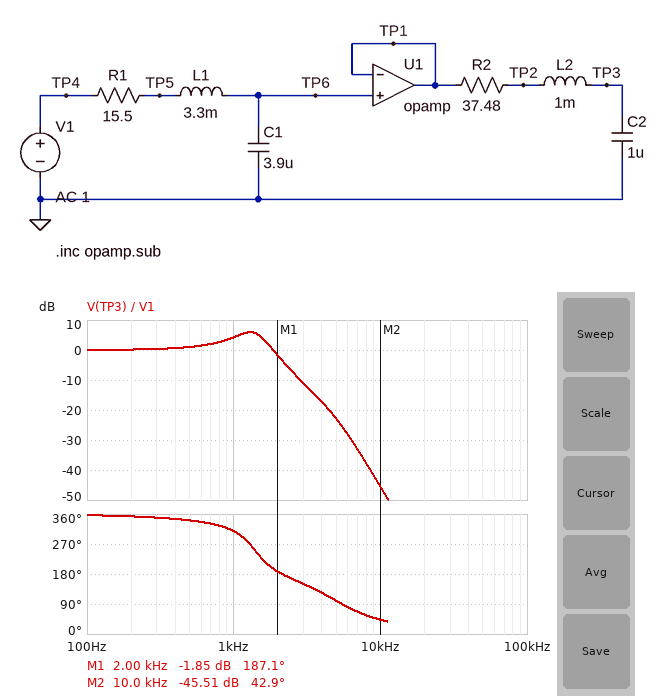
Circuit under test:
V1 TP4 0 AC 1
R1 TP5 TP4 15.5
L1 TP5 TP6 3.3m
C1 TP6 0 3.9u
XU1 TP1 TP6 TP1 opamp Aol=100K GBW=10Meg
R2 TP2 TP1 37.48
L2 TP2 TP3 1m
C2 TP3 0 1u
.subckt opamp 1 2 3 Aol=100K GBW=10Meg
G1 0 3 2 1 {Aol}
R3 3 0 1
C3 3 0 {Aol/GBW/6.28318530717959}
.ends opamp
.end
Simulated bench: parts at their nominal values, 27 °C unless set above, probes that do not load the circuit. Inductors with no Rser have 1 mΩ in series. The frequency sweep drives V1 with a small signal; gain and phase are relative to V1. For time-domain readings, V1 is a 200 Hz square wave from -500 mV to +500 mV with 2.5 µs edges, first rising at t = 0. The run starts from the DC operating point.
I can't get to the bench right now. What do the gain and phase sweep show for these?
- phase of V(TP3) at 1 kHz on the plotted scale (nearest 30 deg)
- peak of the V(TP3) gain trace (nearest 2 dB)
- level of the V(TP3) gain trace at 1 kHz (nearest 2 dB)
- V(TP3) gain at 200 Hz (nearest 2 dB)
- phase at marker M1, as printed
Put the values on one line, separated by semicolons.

300 deg; 6 dB; 4 dB; 0 dB; 187.1 deg
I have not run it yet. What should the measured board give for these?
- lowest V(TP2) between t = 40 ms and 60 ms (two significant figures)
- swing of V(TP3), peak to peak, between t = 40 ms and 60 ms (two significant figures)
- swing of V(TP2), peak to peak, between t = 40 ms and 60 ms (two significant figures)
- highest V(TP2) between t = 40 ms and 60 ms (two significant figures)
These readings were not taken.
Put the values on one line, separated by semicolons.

-900 mV; 1.9 V; 1.8 V; 900 mV
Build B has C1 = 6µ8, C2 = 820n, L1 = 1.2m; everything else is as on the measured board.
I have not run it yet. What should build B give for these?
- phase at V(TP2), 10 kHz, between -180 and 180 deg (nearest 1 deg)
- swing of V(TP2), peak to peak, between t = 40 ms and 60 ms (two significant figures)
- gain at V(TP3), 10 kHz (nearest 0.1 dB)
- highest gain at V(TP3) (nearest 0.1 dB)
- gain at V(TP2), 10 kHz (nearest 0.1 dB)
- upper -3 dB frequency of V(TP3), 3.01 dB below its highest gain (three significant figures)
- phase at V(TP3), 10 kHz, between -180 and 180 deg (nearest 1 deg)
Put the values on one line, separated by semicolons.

-127 deg; 1.2 V; -39.5 dB; 0.6 dB; -32.5 dB; 2.04 kHz; 53 deg
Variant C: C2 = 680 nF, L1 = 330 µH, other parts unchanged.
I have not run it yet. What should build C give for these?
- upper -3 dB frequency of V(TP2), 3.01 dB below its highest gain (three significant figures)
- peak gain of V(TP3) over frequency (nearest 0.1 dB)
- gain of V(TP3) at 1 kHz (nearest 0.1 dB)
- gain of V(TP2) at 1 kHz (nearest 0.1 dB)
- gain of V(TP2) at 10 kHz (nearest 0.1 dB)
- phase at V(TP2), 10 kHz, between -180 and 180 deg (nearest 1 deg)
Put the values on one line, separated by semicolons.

2.82 kHz; 0 dB; -0.1 dB; -0.3 dB; -17.7 dB; -94 deg
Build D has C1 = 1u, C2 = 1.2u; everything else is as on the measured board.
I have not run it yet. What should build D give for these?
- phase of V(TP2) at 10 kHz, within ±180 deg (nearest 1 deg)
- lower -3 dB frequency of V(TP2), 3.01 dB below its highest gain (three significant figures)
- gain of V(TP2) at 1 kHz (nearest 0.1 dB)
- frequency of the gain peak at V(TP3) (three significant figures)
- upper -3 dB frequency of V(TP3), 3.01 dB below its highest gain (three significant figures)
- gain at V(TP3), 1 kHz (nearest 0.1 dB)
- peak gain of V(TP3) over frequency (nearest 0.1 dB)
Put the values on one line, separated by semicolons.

-138 deg; 2.13 kHz; 0.8 dB; 2.71 kHz; 3.06 kHz; 1.2 dB; 11.4 dB
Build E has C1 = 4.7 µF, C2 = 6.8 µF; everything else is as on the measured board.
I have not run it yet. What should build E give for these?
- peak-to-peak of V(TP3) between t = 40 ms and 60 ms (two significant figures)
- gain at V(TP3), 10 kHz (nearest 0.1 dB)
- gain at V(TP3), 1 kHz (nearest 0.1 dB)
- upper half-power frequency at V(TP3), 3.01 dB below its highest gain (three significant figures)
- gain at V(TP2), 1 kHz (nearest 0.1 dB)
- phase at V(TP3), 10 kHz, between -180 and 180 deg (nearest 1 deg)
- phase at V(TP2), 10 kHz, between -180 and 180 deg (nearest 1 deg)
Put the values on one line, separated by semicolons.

1.1 V; -65.3 dB; -0.5 dB; 1.36 kHz; -3.2 dB; 36 deg; -144 deg
